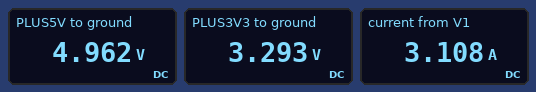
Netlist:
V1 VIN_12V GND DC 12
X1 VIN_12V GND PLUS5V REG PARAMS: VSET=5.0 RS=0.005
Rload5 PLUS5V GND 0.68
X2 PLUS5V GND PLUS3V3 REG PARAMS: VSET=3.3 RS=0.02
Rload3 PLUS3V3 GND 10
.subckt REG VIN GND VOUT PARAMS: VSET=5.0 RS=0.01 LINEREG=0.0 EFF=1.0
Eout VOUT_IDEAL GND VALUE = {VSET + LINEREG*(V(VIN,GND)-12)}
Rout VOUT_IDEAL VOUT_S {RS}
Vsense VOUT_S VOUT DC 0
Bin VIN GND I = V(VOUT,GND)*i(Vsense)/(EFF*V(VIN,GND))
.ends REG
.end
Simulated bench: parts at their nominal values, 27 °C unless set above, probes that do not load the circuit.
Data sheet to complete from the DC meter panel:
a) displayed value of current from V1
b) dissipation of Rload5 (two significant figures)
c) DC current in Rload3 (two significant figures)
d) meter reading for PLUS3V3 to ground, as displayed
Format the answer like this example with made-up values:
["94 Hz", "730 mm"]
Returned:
["3.108 A", "36 W", "330 mA", "3.293 V"]
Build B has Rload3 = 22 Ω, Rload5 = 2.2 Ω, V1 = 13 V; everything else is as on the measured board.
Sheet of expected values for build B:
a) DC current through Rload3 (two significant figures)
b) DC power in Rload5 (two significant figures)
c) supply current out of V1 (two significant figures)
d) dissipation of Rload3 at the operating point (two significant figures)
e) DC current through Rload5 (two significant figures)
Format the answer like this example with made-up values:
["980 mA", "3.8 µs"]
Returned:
["150 mA", "11 W", "910 mA", "490 mW", "2.3 A"]
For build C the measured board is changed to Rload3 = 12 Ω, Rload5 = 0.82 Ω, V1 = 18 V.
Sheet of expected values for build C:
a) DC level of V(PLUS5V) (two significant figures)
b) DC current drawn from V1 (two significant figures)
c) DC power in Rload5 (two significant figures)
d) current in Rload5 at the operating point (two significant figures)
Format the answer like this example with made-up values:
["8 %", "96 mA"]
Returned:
["5.0 V", "1.7 A", "30 W", "6.1 A"]
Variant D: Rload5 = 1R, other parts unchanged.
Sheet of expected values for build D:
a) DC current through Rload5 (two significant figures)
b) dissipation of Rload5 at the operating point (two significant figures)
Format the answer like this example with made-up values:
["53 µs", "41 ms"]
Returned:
["5.0 A", "25 W"]
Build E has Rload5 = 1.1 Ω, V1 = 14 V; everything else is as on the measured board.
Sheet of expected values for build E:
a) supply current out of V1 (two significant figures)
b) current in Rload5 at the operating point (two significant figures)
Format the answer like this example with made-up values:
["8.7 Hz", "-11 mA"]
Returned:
["1.7 A", "4.5 A"]
